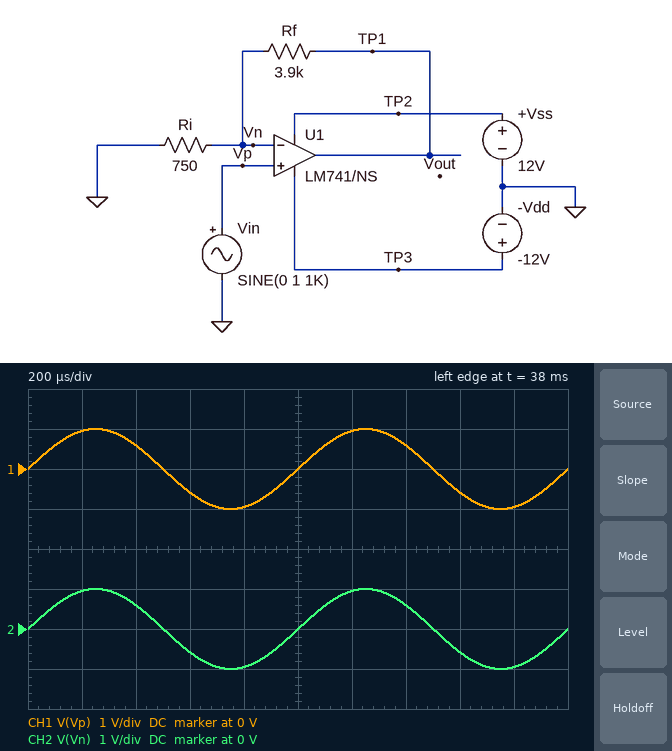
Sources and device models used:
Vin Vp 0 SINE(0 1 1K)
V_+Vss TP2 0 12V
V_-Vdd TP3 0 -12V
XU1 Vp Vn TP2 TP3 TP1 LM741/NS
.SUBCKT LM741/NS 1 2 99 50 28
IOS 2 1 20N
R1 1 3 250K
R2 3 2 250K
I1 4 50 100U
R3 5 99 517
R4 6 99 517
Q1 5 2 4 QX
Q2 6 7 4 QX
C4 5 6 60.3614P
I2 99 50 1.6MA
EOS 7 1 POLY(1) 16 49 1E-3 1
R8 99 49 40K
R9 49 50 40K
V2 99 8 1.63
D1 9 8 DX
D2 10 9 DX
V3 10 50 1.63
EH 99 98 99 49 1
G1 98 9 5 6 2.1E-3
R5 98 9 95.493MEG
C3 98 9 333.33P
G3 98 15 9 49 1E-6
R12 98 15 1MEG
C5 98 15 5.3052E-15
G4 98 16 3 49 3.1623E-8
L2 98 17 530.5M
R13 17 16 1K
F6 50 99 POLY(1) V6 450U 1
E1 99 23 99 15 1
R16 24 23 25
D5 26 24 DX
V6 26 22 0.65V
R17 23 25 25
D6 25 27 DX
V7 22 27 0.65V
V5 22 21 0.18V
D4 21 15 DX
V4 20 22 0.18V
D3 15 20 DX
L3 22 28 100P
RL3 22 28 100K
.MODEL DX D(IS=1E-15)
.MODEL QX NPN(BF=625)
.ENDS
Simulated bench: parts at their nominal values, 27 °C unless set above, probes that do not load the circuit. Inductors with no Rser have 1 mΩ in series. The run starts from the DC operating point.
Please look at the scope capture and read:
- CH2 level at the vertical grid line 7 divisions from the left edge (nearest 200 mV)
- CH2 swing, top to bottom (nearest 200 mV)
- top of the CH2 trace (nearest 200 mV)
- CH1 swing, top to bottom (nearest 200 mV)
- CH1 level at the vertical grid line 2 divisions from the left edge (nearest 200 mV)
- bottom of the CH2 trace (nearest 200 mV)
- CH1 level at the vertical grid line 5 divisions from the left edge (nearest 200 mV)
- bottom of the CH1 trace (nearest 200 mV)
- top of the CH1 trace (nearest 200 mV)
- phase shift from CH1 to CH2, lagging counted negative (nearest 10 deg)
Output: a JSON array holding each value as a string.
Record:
["600 mV", "2.0 V", "1.0 V", "2.0 V", "600 mV", "-1.0 V", "0 V", "-1.0 V", "1.0 V", "0 deg"]
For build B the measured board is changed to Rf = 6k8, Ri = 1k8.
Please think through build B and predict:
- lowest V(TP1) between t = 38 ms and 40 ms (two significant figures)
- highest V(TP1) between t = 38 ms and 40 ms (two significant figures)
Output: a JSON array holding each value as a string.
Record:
["-4.8 V", "4.8 V"]
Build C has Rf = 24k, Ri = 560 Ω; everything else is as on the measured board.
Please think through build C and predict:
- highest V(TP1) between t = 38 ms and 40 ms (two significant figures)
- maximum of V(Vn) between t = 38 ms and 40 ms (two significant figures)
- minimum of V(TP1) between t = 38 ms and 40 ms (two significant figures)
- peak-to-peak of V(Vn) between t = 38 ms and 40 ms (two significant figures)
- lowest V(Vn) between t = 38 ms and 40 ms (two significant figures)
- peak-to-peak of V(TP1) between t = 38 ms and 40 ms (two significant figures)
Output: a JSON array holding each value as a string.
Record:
["11 V", "250 mV", "-11 V", "500 mV", "-250 mV", "22 V"]
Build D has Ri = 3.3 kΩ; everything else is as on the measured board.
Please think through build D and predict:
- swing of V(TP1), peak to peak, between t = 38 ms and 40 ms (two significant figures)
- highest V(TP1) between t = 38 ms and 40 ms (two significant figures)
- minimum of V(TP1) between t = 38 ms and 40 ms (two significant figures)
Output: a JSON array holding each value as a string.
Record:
["4.4 V", "2.2 V", "-2.2 V"]
